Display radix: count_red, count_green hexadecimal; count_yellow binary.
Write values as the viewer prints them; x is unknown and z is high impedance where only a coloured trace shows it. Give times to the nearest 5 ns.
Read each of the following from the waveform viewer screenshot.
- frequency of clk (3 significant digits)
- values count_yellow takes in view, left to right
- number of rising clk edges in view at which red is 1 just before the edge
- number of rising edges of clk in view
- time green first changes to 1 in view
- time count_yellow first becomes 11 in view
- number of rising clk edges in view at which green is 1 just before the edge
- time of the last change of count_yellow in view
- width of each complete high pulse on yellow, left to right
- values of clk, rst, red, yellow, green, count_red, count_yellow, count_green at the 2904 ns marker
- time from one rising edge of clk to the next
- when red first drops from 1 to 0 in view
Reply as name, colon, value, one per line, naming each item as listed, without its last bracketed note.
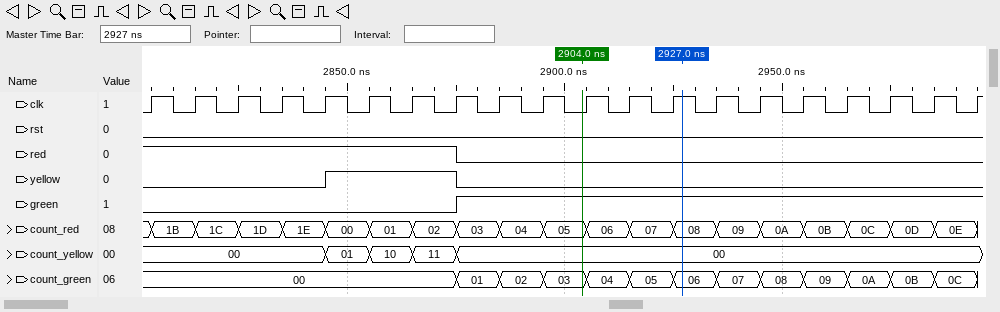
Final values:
frequency of clk: 100 MHz
values count_yellow takes in view, left to right: 00, 01, 10, 11, 00
number of rising clk edges in view at which red is 1 just before the edge: 8
number of rising edges of clk in view: 20
time green first changes to 1 in view: 2875 ns
time count_yellow first becomes 11 in view: 2865 ns
number of rising clk edges in view at which green is 1 just before the edge: 12
time of the last change of count_yellow in view: 2875 ns
width of each complete high pulse on yellow, left to right: 30 ns
values of clk, rst, red, yellow, green, count_red, count_yellow, count_green at the 2904 ns marker: clk=0, rst=0, red=0, yellow=0, green=1, count_red=05, count_yellow=00, count_green=03
time from one rising edge of clk to the next: 10 ns
when red first drops from 1 to 0 in view: 2875 ns
